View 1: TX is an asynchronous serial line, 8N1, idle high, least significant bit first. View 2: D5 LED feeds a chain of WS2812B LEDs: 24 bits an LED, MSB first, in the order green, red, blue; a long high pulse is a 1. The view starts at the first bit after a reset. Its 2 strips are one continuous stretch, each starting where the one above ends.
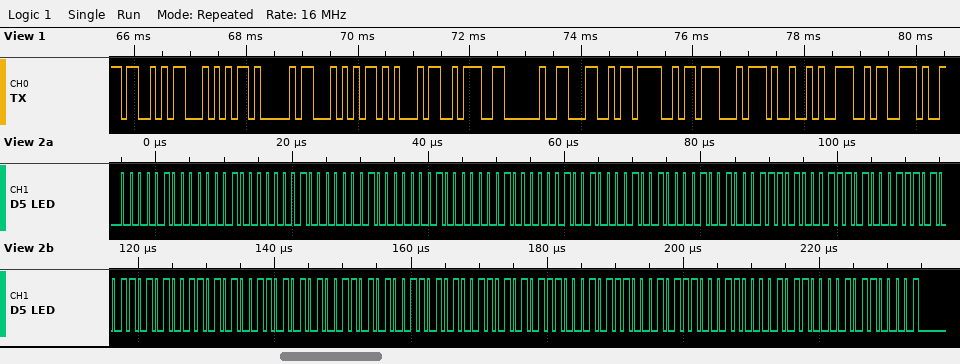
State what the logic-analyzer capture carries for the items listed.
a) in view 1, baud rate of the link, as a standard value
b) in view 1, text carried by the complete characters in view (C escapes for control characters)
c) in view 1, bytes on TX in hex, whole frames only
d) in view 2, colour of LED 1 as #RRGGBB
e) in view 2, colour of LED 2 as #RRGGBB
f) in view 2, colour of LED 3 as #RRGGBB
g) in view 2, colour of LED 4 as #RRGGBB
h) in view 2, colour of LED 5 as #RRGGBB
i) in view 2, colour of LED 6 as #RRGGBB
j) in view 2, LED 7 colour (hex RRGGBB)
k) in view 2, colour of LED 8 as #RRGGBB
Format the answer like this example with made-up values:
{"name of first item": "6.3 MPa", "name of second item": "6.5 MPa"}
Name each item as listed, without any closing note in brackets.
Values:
{"in view 1, baud rate of the link, as a standard value": "9600 baud", "in view 1, text carried by the complete characters in view": "\"STATE: LOGIN.\"", "in view 1, bytes on TX in hex, whole frames only": "0x53 0x54 0x41 0x54 0x45 0x3A 0x20 0x4C 0x4F 0x47 0x49 0x4E 0x2E", "in view 2, colour of LED 1 as #RRGGBB": "#040404", "in view 2, colour of LED 2 as #RRGGBB": "#040404", "in view 2, colour of LED 3 as #RRGGBB": "#090909", "in view 2, colour of LED 4 as #RRGGBB": "#1D1D1D", "in view 2, colour of LED 5 as #RRGGBB": "#353535", "in view 2, colour of LED 6 as #RRGGBB": "#4D4D4D", "in view 2, LED 7 colour": "#5C5C5C", "in view 2, colour of LED 8 as #RRGGBB": "#616161"}
